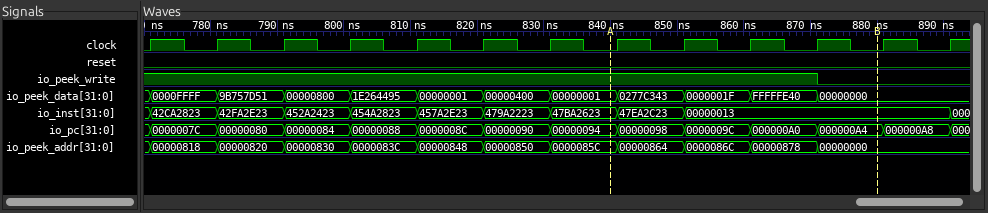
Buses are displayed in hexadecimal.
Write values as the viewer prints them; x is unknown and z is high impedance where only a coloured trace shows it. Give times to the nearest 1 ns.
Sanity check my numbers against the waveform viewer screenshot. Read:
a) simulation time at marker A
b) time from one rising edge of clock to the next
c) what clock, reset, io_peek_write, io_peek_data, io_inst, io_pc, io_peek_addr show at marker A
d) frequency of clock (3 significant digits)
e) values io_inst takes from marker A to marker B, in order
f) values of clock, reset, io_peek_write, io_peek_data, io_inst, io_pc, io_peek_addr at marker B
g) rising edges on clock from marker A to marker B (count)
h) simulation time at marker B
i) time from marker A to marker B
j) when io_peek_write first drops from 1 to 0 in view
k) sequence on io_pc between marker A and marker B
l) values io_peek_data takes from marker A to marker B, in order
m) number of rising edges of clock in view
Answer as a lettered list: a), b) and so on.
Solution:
a) 840 ns
b) 10 ns
c) clock=0, reset=0, io_peek_write=1, io_peek_data=00000001, io_inst=47BA2623, io_pc=00000094, io_peek_addr=0000085C
d) 100 MHz
e) 47BA2623, 47EA2C23, 00000013
f) clock=0, reset=0, io_peek_write=0, io_peek_data=00000000, io_inst=00000013, io_pc=000000A4, io_peek_addr=00000000
g) 4
h) 880 ns
i) 40 ns
j) 871 ns
k) 00000094, 00000098, 0000009C, 000000A0, 000000A4
l) 00000001, 0277C343, 0000001F, FFFFFE40, 00000000
m) 13
